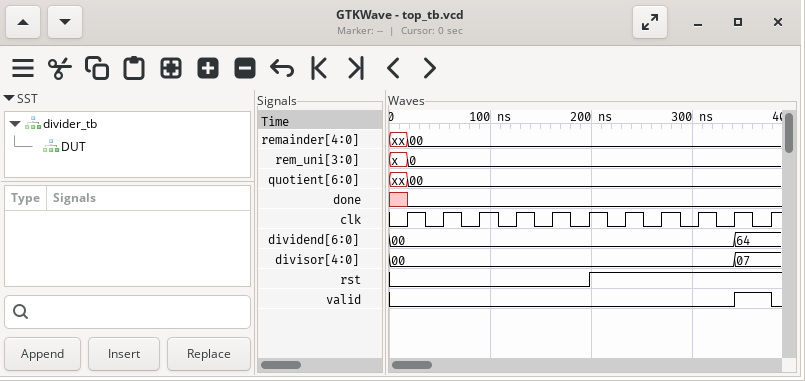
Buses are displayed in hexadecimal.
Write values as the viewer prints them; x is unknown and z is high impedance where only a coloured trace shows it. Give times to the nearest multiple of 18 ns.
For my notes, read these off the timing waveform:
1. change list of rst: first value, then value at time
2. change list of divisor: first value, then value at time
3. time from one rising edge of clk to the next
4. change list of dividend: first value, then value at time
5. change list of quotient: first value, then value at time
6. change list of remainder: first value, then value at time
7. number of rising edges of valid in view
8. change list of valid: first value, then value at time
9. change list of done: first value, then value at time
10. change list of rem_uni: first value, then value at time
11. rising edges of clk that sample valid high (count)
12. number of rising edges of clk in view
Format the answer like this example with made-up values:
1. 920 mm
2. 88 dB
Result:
1. 0, 1 at 198 ns
2. 00, 07 at 342 ns
3. 36 ns
4. 00, 64 at 342 ns
5. xx, 00 at 18 ns
6. xx, 00 at 18 ns
7. 1
8. 0, 1 at 342 ns, 0 at 378 ns
9. x, 0 at 18 ns
10. x, 0 at 18 ns
11. 1
12. 11
